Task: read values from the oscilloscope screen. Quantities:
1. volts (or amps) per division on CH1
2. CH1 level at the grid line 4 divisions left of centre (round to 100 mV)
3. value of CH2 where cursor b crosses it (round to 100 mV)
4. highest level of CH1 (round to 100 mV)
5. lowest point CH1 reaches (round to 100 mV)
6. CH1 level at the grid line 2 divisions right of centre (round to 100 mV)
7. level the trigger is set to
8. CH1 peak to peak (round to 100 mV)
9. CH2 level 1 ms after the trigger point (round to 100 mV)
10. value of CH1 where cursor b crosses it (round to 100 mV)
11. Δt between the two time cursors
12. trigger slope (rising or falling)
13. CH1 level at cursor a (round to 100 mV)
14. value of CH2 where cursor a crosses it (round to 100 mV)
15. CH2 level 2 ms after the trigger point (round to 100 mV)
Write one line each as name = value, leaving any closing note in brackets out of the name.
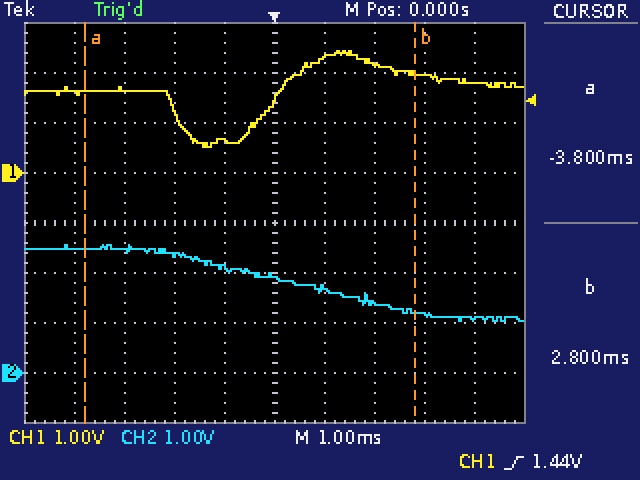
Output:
volts (or amps) per division on CH1 = 1 V
CH1 level at the grid line 4 divisions left of centre = 1.6 V
value of CH2 where cursor b crosses it = 1.2 V
highest level of CH1 = 2.4 V
lowest point CH1 reaches = 500 mV
CH1 level at the grid line 2 divisions right of centre = 2.2 V
level the trigger is set to = 1.44 V
CH1 peak to peak = 1.9 V
CH2 level 1 ms after the trigger point = 1.7 V
value of CH1 where cursor b crosses it = 2.0 V
Δt between the two time cursors = 6.6 ms
trigger slope = rising
CH1 level at cursor a = 1.6 V
value of CH2 where cursor a crosses it = 2.5 V
CH2 level 2 ms after the trigger point = 1.4 V
